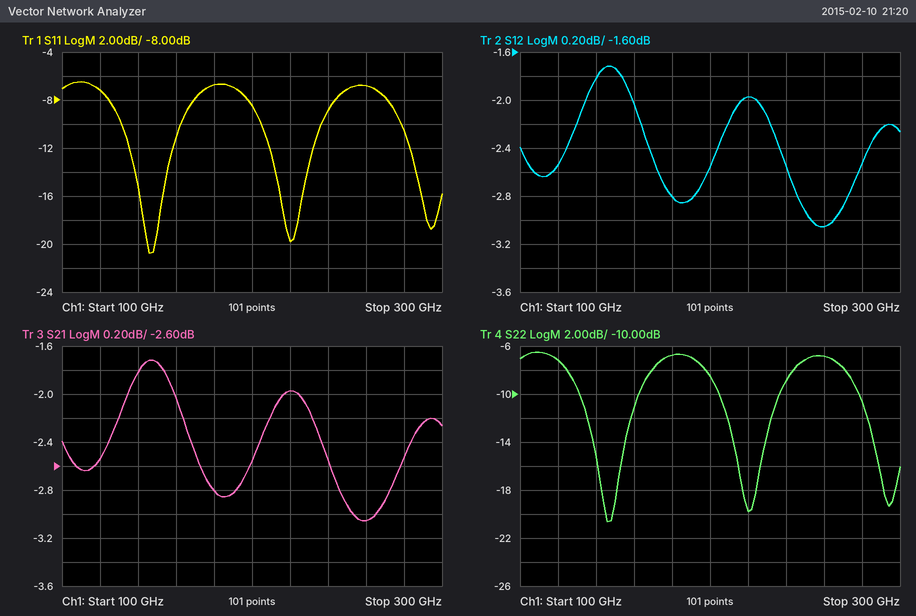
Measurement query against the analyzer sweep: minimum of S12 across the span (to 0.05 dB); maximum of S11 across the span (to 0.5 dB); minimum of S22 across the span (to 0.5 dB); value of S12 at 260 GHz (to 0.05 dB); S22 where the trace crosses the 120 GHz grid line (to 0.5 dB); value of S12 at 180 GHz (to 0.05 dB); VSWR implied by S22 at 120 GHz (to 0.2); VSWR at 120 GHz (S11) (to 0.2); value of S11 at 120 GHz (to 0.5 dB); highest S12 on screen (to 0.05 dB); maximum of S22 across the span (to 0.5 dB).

-3.05 dB
-6.5 dB
-20.5 dB
-3.05 dB
-7.0 dB
-2.80 dB
2.6
2.6
-7.0 dB
-1.70 dB
-6.5 dB
